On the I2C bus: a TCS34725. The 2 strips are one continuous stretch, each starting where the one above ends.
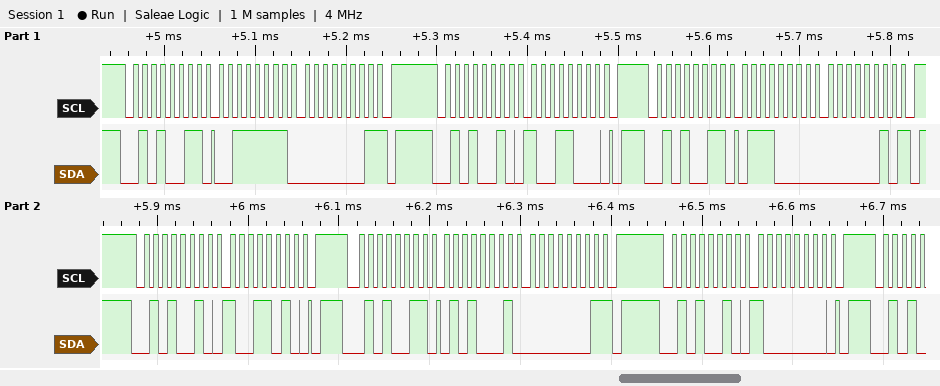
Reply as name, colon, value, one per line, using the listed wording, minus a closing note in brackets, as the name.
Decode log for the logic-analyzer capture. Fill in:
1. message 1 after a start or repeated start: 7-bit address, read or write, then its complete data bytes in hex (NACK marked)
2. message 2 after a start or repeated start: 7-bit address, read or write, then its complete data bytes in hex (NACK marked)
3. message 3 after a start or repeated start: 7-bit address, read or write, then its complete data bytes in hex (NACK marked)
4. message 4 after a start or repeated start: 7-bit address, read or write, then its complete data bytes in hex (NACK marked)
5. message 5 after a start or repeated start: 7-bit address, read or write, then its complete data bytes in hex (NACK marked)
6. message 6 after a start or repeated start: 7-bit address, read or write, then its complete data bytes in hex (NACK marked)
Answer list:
message 1 after a start or repeated start: 7-bit address, read or write, then its complete data bytes in hex: 0x29 read: 3F 01 NACK
message 2 after a start or repeated start: 7-bit address, read or write, then its complete data bytes in hex: 0x29 write: 98
message 3 after a start or repeated start: 7-bit address, read or write, then its complete data bytes in hex: 0x29 read: 70 02 NACK
message 4 after a start or repeated start: 7-bit address, read or write, then its complete data bytes in hex: 0x29 write: 9A
message 5 after a start or repeated start: 7-bit address, read or write, then its complete data bytes in hex: 0x29 read: 51 01 NACK
message 6 after a start or repeated start: 7-bit address, read or write, then its complete data bytes in hex: 0x29 write: 80
